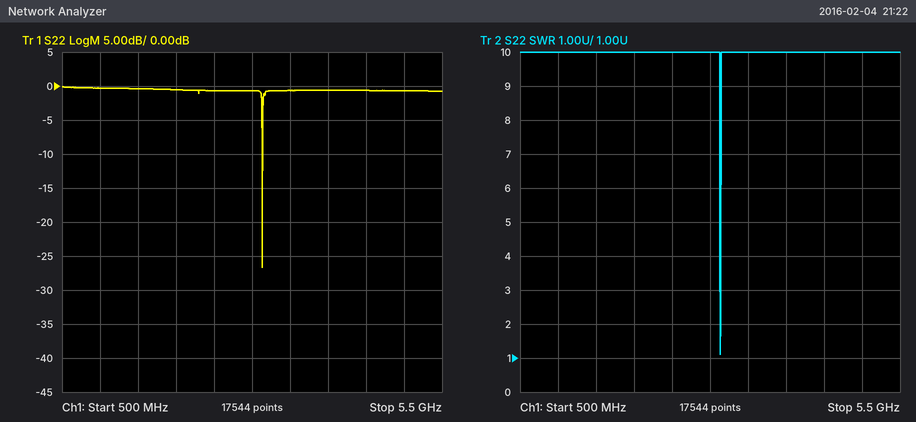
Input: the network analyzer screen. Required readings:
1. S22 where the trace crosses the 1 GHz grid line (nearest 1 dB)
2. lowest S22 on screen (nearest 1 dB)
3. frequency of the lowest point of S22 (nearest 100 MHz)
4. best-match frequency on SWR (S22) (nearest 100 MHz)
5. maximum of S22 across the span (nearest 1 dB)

0 dB
-27 dB
3.1 GHz
3.1 GHz
0 dB
